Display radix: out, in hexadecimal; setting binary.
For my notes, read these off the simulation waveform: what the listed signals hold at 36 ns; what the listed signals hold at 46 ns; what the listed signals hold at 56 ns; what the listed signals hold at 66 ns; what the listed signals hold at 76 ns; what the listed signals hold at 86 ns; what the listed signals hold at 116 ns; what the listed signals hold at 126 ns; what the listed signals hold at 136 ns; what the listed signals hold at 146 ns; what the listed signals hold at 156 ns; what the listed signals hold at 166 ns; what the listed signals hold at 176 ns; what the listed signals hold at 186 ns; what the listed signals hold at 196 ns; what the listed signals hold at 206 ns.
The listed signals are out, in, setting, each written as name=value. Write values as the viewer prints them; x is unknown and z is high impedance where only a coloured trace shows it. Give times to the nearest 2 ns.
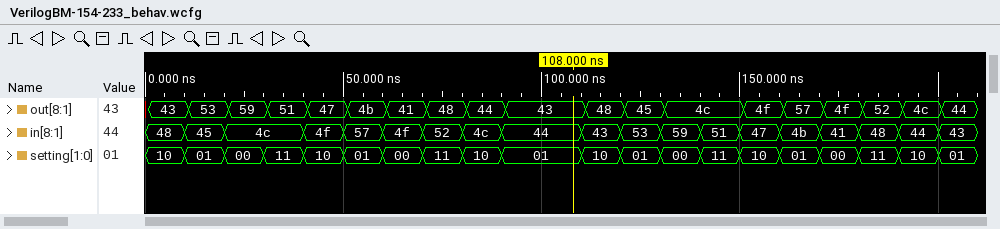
out=51, in=4c, setting=11
out=47, in=4f, setting=10
out=4b, in=57, setting=01
out=41, in=4f, setting=00
out=48, in=52, setting=11
out=44, in=4c, setting=10
out=48, in=43, setting=10
out=45, in=53, setting=01
out=4c, in=59, setting=00
out=4c, in=51, setting=11
out=4f, in=47, setting=10
out=57, in=4b, setting=01
out=4f, in=41, setting=00
out=52, in=48, setting=11
out=4c, in=44, setting=10
out=44, in=43, setting=01
